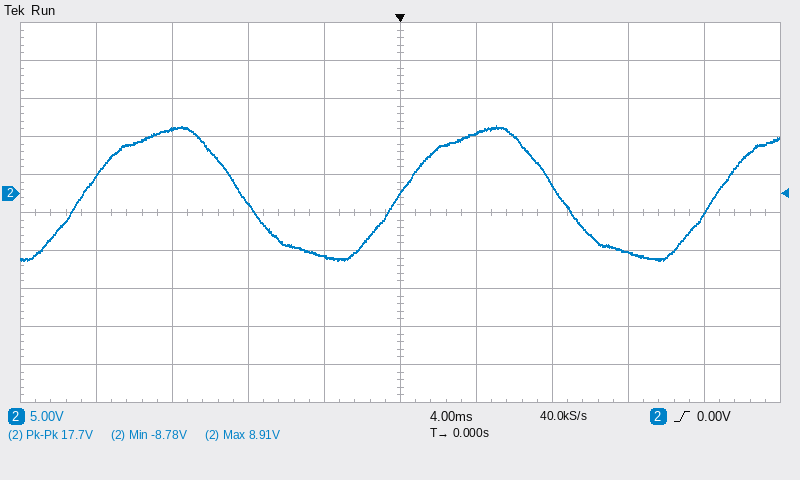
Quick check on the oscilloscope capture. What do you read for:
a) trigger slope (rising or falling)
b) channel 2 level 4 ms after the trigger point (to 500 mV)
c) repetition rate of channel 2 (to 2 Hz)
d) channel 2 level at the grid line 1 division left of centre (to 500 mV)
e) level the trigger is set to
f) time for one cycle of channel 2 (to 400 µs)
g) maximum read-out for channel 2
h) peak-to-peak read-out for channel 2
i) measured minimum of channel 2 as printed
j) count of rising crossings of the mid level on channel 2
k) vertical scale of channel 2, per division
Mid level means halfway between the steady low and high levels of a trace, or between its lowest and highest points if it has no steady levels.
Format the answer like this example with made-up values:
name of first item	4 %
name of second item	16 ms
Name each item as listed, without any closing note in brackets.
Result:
trigger slope	rising
channel 2 level 4 ms after the trigger point	8.0 V
repetition rate of channel 2	60 Hz
channel 2 level at the grid line 1 division left of centre	-8.5 V
level the trigger is set to	0.00 V
time for one cycle of channel 2	16.8 ms
maximum read-out for channel 2	8.91 V
peak-to-peak read-out for channel 2	17.7 V
measured minimum of channel 2 as printed	-8.78 V
count of rising crossings of the mid level on channel 2	3
vertical scale of channel 2, per division	5 V
